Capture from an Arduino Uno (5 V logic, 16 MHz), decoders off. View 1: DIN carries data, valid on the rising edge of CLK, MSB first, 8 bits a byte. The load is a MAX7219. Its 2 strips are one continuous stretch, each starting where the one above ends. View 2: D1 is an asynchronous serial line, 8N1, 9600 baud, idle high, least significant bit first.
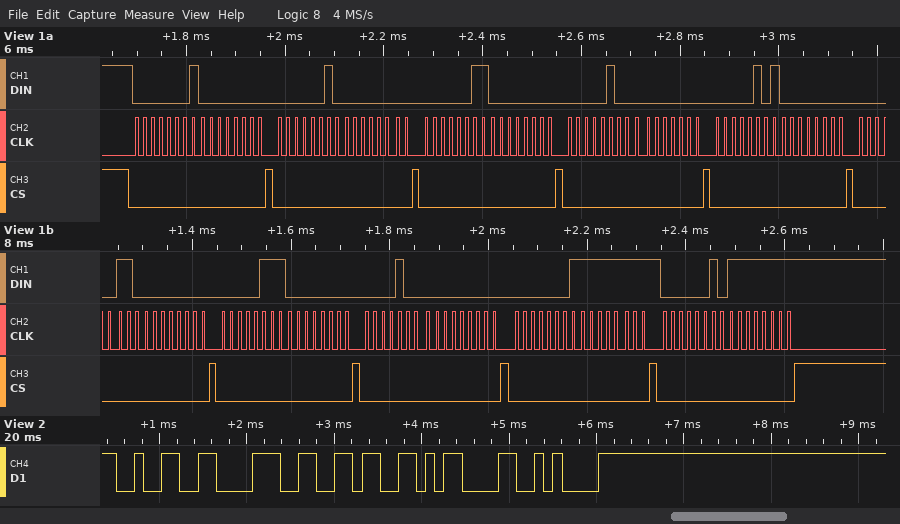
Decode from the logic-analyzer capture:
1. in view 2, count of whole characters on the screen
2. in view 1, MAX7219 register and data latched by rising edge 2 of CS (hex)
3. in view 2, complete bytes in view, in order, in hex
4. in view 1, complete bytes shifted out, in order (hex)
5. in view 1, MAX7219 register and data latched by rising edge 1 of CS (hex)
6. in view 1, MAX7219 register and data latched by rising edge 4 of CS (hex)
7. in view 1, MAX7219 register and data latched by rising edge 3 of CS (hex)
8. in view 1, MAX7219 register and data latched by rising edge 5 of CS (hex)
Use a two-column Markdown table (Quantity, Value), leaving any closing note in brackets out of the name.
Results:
| Quantity | Value |
|---|---|
| in view 2, count of whole characters on the screen | 5 |
| in view 1, MAX7219 register and data latched by rising edge 2 of CS | register 0x2, data 0x00 |
| in view 2, complete bytes in view, in order, in hex | 0x32 0x38 0x36 0x0D 0x0A |
| in view 1, complete bytes shifted out, in order | 01 00 02 00 03 00 04 00 05 00 06 00 07 00 08 00 01 FF 02 FF |
| in view 1, MAX7219 register and data latched by rising edge 1 of CS | register 0x1, data 0x00 |
| in view 1, MAX7219 register and data latched by rising edge 4 of CS | register 0x4, data 0x00 |
| in view 1, MAX7219 register and data latched by rising edge 3 of CS | register 0x3, data 0x00 |
| in view 1, MAX7219 register and data latched by rising edge 5 of CS | register 0x5, data 0x00 |
